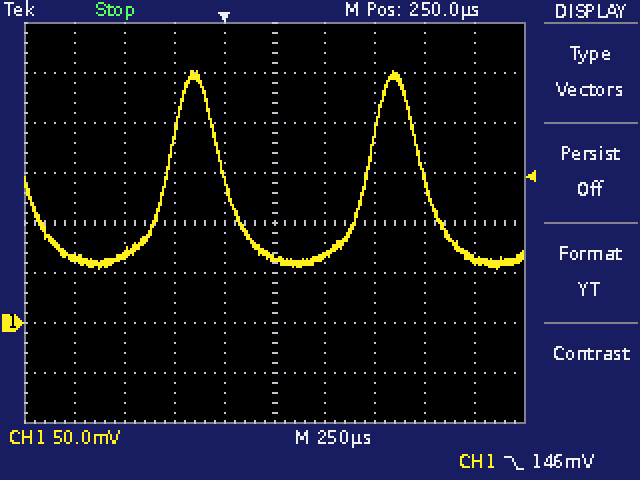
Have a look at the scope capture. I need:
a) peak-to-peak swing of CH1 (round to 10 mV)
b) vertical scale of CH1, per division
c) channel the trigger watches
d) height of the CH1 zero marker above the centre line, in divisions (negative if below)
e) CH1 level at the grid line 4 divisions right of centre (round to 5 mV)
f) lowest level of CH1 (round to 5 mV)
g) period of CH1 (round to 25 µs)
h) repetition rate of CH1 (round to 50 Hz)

200 mV
50 mV
CH1
-2.0 div
65 mV
55 mV
1.000 ms
1.00 kHz
